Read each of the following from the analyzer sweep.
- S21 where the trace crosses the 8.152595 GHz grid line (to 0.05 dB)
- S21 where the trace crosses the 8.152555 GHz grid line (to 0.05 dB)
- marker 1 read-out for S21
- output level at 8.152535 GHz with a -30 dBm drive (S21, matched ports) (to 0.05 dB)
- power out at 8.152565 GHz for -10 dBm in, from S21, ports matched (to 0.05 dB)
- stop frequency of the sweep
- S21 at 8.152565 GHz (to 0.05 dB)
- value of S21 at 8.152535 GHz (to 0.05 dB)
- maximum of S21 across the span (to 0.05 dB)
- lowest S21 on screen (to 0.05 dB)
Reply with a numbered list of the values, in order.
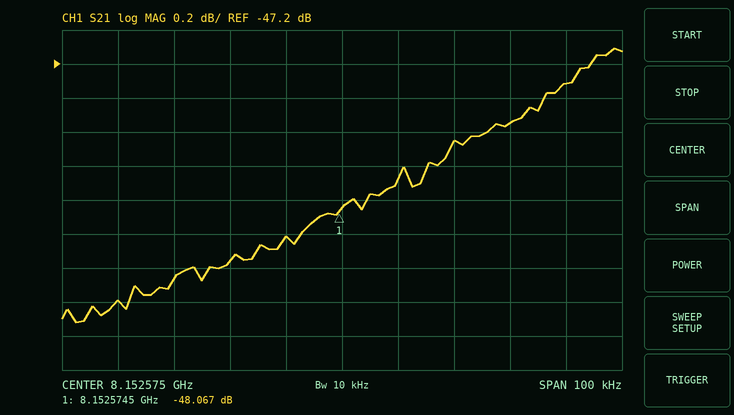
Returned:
1. -47.65 dB
2. -48.35 dB
3. -48.067 dB
4. -78.60 dBm
5. -58.20 dBm
6. 8.152625 GHz
7. -48.20 dB
8. -48.60 dB
9. -47.10 dB
10. -48.70 dB
